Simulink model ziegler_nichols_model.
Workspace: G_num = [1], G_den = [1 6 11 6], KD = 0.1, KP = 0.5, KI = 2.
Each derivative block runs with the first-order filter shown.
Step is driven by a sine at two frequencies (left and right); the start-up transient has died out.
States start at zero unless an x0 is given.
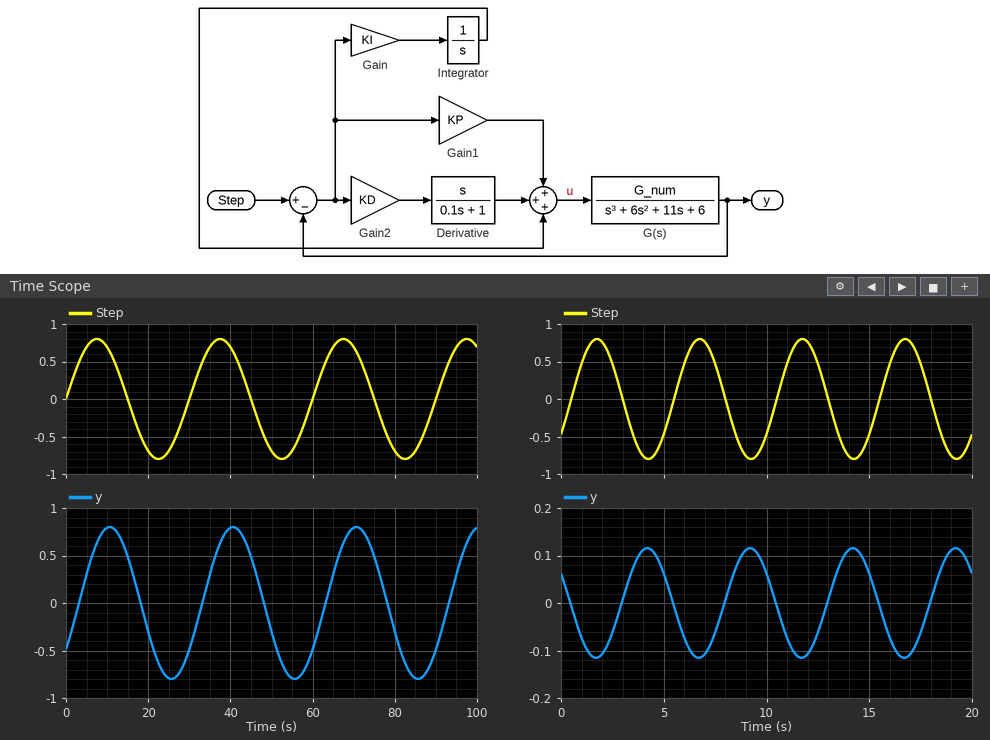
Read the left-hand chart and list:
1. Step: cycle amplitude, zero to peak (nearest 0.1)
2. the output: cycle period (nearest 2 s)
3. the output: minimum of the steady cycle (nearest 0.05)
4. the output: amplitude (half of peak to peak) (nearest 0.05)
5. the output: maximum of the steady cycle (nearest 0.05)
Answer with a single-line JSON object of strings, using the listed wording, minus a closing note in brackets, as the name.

{"Step: cycle amplitude, zero to peak": "0.8", "the output: cycle period": "30 s", "the output: minimum of the steady cycle": "-0.80", "the output: amplitude (half of peak to peak)": "0.80", "the output: maximum of the steady cycle": "0.80"}
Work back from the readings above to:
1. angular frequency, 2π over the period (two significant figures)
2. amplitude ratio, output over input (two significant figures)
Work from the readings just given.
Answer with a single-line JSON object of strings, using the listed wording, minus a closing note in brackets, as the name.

{"angular frequency, 2π over the period": "0.21 rad/s", "amplitude ratio, output over input": "1.0"}
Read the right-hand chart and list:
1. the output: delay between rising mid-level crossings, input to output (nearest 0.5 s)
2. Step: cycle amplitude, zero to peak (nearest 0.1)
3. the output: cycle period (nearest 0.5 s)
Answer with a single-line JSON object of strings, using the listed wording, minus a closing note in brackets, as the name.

{"the output: delay between rising mid-level crossings, input to output": "2.5 s", "Step: cycle amplitude, zero to peak": "0.8", "the output: cycle period": "5.0 s"}
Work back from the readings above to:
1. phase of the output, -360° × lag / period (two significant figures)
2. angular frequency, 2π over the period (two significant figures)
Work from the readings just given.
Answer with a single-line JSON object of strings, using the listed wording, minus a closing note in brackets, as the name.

{"phase of the output, -360° × lag / period": "-180°", "angular frequency, 2π over the period": "1.3 rad/s"}
